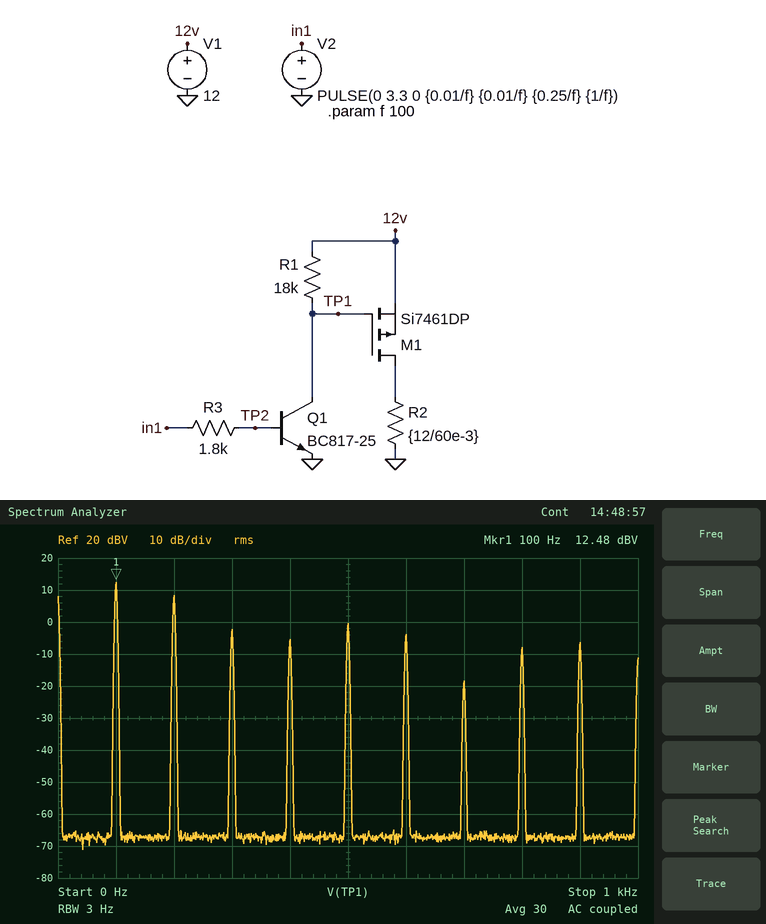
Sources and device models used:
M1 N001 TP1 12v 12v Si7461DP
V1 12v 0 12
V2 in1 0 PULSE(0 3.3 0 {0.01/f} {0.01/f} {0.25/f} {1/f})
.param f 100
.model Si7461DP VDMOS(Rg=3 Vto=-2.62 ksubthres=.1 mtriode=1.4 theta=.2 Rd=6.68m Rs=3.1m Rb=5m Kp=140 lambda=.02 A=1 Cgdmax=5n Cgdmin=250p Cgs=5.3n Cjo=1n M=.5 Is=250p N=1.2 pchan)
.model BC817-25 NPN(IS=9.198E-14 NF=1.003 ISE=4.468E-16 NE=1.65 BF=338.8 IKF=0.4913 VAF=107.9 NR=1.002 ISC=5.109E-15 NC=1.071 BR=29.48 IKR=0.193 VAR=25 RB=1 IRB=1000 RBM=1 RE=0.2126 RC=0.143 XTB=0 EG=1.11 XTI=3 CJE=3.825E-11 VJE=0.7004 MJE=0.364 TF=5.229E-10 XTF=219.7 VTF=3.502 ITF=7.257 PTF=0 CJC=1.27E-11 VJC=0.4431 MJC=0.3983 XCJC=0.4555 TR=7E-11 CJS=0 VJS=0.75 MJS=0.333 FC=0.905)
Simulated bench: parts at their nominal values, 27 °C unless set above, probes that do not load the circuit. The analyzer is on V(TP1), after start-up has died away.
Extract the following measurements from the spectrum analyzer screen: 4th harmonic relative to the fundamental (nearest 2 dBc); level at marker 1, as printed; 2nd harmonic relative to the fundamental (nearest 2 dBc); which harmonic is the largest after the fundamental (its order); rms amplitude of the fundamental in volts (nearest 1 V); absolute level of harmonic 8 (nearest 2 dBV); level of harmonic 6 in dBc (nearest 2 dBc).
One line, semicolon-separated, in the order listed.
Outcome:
-18 dBc; 12.48 dBV; -4 dBc; 2; 4 V; -8 dBV; -16 dBc
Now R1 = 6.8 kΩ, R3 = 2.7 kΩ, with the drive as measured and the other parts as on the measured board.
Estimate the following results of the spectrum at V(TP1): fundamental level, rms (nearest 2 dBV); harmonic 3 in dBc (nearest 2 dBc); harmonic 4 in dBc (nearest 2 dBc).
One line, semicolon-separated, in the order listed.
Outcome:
12 dBV; -12 dBc; -20 dBc
